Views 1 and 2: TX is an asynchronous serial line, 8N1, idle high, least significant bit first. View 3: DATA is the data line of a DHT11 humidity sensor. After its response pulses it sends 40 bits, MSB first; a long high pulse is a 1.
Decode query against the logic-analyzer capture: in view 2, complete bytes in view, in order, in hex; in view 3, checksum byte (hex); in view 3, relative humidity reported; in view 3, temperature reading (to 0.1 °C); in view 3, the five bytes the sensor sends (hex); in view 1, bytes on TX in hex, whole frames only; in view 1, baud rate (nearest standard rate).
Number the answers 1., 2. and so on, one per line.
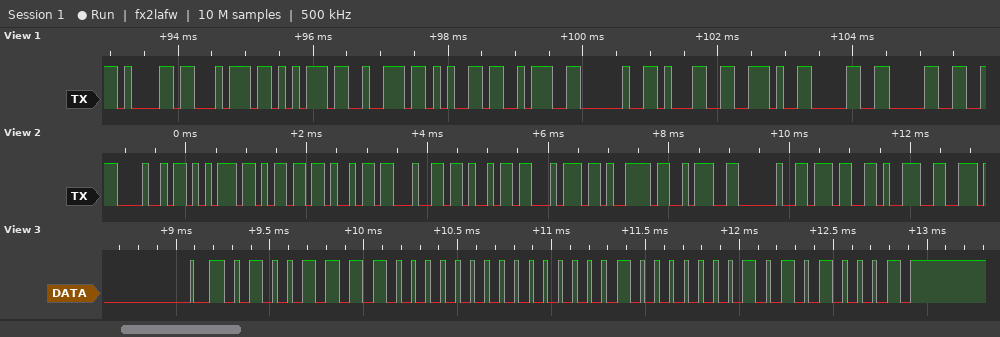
1. 48 75 6D 69 64 69 74 79 3A 20 37 39
2. 0x51
3. 79 %
4. 1.1 °C
5. 4F 00 01 01 51
6. 61 74 75 72 65 3A 20 31 2E 30 30
7. 9600 baud
